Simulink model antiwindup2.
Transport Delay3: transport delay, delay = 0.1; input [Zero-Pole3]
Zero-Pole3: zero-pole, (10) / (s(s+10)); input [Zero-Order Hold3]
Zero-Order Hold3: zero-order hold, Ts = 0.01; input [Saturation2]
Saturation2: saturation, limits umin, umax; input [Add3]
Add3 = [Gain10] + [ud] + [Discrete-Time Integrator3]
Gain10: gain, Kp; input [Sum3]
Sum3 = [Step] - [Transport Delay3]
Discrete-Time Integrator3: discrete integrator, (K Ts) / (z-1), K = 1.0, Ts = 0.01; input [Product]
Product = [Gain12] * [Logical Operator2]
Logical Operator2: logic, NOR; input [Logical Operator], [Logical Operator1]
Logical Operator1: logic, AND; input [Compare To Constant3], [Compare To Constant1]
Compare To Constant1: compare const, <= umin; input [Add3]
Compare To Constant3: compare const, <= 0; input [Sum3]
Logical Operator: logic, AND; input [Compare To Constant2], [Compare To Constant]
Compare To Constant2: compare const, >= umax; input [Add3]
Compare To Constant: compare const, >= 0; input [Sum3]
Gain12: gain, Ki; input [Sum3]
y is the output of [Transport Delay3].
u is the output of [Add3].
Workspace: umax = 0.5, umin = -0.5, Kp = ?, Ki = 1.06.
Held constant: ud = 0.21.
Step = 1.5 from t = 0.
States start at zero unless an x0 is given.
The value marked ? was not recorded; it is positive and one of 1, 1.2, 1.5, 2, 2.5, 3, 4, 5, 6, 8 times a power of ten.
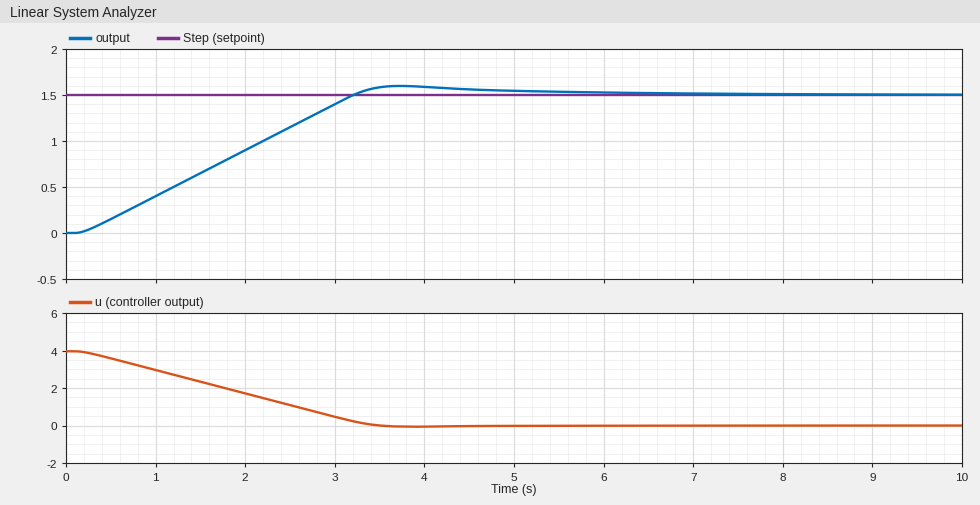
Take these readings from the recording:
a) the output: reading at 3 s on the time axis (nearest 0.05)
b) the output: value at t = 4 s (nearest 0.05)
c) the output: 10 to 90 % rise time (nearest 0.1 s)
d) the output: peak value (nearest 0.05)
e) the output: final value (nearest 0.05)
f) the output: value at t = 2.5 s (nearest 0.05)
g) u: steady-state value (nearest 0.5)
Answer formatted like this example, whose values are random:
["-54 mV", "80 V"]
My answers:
["1.40", "1.60", "2.4 s", "1.60", "1.50", "1.15", "0.0"]
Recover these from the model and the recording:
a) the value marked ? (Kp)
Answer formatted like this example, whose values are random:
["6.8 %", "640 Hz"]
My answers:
["2.5"]
